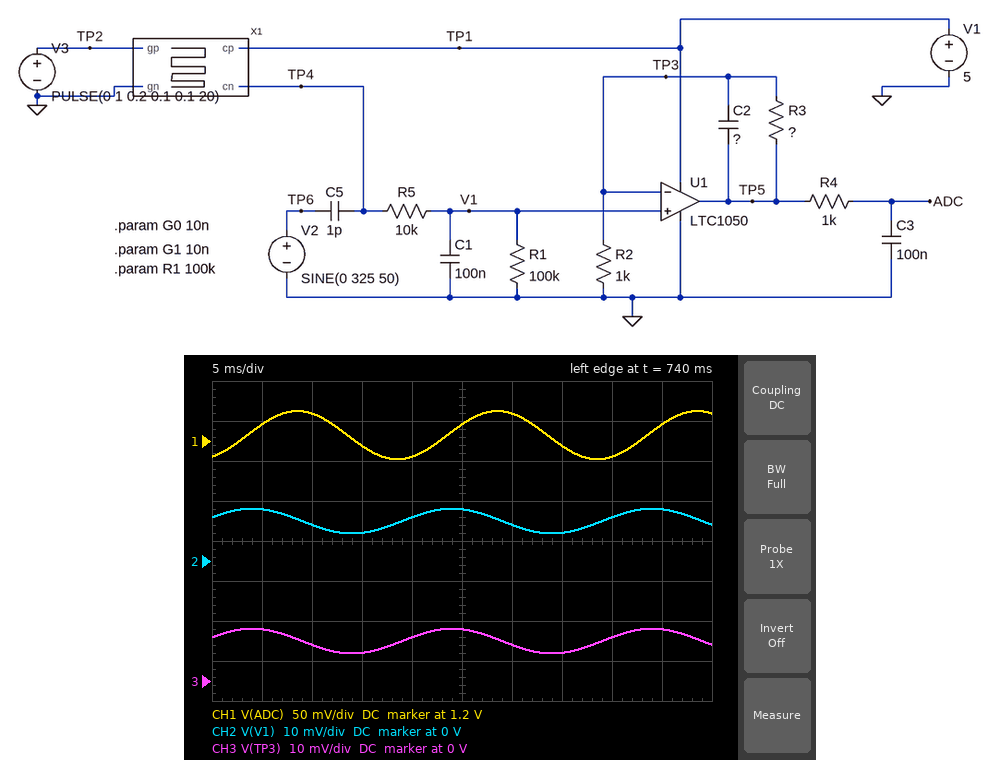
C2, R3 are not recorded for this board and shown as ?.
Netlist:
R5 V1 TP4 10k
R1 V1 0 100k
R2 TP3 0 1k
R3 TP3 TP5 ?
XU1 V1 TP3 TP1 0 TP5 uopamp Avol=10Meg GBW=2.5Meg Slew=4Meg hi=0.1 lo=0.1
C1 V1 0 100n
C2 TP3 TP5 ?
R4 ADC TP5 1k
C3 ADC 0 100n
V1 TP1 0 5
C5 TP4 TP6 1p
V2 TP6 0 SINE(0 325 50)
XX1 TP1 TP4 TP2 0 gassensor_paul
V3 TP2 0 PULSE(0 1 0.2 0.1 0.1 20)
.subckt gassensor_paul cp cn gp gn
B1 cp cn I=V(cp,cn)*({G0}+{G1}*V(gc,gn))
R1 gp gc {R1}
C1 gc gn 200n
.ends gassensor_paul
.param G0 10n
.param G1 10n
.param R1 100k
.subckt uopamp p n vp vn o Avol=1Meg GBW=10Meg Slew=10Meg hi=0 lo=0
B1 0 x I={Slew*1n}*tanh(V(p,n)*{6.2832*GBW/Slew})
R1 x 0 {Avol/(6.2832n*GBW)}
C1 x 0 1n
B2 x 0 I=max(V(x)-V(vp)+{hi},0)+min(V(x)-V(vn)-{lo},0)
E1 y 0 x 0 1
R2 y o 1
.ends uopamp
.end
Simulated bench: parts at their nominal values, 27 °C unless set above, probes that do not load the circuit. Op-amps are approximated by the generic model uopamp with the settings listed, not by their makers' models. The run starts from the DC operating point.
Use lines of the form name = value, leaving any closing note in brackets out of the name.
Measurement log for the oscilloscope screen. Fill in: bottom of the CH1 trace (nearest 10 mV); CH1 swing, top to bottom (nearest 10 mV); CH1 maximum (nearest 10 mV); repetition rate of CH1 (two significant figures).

bottom of the CH1 trace = 1.18 V
CH1 swing, top to bottom = 60 mV
CH1 maximum = 1.24 V
repetition rate of CH1 = 50 Hz
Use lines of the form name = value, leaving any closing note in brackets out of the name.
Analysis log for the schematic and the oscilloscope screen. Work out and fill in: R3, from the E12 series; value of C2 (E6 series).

R3, from the E12 series = 120 kΩ
value of C2 = 330 nF
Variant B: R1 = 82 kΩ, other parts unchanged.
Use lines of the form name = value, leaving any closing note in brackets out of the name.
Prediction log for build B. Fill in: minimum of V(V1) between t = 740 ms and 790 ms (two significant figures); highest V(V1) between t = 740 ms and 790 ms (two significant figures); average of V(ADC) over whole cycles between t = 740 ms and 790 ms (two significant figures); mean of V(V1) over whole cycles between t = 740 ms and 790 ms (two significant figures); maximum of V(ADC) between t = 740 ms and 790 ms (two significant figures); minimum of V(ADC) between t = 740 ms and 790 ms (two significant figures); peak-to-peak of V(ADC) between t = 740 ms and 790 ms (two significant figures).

minimum of V(V1) between t = 740 ms and 790 ms = 5.2 mV
highest V(V1) between t = 740 ms and 790 ms = 11 mV
average of V(ADC) over whole cycles between t = 740 ms and 790 ms = 990 mV
mean of V(V1) over whole cycles between t = 740 ms and 790 ms = 8.2 mV
maximum of V(ADC) between t = 740 ms and 790 ms = 1.0 V
minimum of V(ADC) between t = 740 ms and 790 ms = 960 mV
peak-to-peak of V(ADC) between t = 740 ms and 790 ms = 59 mV
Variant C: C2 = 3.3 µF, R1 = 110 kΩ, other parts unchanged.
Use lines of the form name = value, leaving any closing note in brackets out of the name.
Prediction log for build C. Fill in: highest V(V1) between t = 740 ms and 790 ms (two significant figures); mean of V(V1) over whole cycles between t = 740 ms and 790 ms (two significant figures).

highest V(V1) between t = 740 ms and 790 ms = 14 mV
mean of V(V1) over whole cycles between t = 740 ms and 790 ms = 11 mV
